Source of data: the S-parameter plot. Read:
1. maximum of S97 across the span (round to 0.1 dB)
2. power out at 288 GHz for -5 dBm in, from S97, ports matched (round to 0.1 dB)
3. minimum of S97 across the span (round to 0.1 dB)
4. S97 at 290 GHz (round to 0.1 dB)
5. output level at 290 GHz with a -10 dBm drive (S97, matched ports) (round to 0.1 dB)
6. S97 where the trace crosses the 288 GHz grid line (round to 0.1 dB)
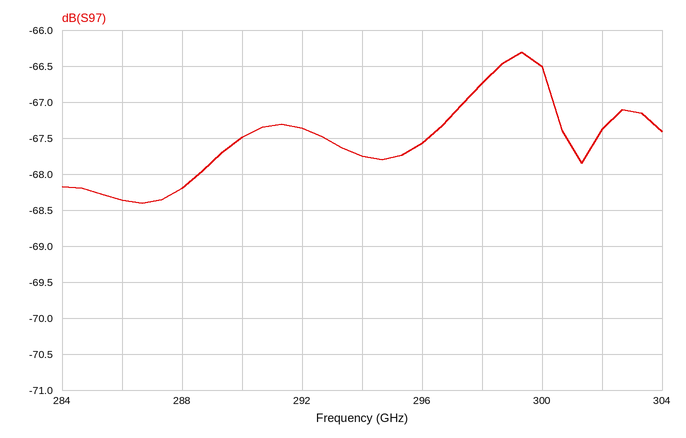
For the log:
-66.3 dB
-73.2 dBm
-68.4 dB
-67.5 dB
-77.5 dBm
-68.2 dB
